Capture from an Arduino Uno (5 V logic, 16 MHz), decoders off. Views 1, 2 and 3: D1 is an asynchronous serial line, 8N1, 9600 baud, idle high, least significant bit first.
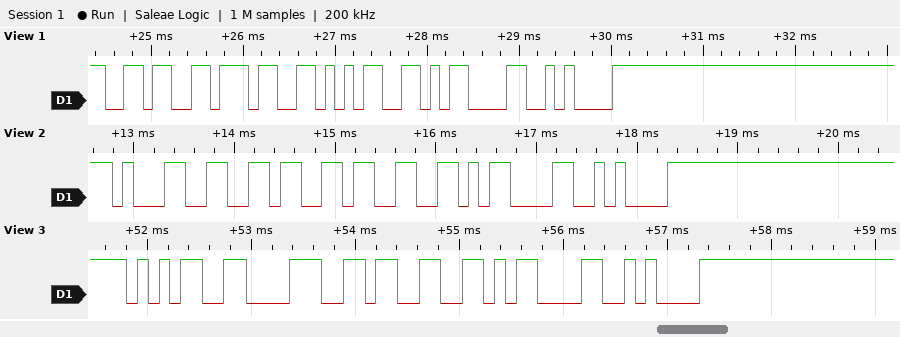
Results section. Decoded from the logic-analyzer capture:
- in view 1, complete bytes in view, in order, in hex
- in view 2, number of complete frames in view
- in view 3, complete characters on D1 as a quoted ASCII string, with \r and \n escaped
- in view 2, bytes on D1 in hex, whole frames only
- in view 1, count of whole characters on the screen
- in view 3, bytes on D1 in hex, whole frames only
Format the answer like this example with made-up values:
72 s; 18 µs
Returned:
36 37 35 0D 0A; 5; "583\r\n"; 31 36 33 0D 0A; 5; 0x35 0x38 0x33 0x0D 0x0A
